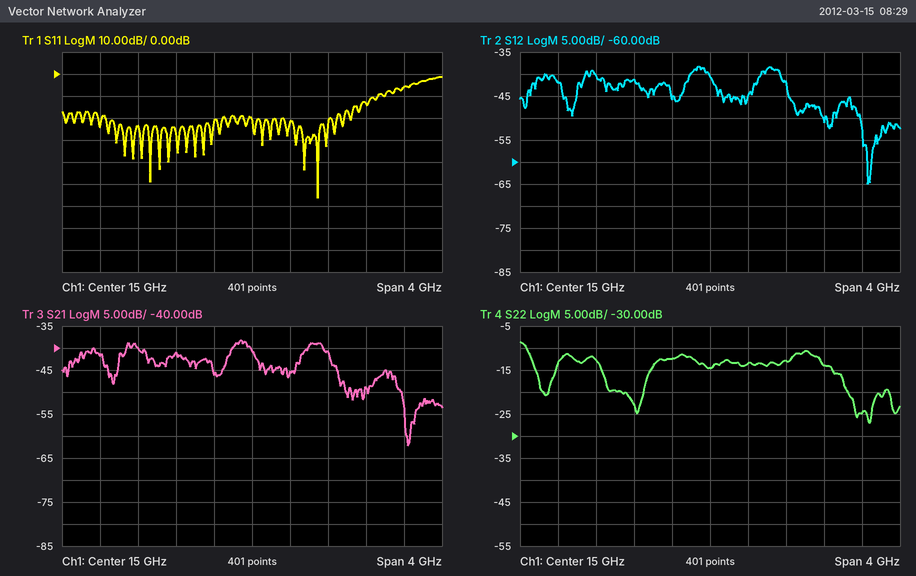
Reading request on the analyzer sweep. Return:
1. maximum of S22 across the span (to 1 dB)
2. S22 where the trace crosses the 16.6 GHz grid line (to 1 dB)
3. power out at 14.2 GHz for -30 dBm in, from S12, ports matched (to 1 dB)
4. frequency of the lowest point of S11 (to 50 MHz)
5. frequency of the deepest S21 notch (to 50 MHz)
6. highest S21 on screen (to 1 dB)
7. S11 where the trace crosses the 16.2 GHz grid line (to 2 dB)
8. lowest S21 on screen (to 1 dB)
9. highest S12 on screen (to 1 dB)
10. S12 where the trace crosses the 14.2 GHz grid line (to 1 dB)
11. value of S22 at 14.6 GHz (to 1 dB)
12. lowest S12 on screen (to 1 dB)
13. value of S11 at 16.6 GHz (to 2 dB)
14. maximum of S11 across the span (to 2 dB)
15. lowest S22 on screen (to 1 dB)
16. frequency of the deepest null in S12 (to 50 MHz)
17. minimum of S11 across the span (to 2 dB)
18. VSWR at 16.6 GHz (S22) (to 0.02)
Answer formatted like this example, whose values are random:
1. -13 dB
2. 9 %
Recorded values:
1. -9 dB
2. -25 dB
3. -71 dBm
4. 15.70 GHz
5. 16.65 GHz
6. -38 dB
7. -14 dB
8. -62 dB
9. -38 dB
10. -41 dB
11. -12 dB
12. -65 dB
13. -6 dB
14. -2 dB
15. -27 dB
16. 16.65 GHz
17. -56 dB
18. 1.12
